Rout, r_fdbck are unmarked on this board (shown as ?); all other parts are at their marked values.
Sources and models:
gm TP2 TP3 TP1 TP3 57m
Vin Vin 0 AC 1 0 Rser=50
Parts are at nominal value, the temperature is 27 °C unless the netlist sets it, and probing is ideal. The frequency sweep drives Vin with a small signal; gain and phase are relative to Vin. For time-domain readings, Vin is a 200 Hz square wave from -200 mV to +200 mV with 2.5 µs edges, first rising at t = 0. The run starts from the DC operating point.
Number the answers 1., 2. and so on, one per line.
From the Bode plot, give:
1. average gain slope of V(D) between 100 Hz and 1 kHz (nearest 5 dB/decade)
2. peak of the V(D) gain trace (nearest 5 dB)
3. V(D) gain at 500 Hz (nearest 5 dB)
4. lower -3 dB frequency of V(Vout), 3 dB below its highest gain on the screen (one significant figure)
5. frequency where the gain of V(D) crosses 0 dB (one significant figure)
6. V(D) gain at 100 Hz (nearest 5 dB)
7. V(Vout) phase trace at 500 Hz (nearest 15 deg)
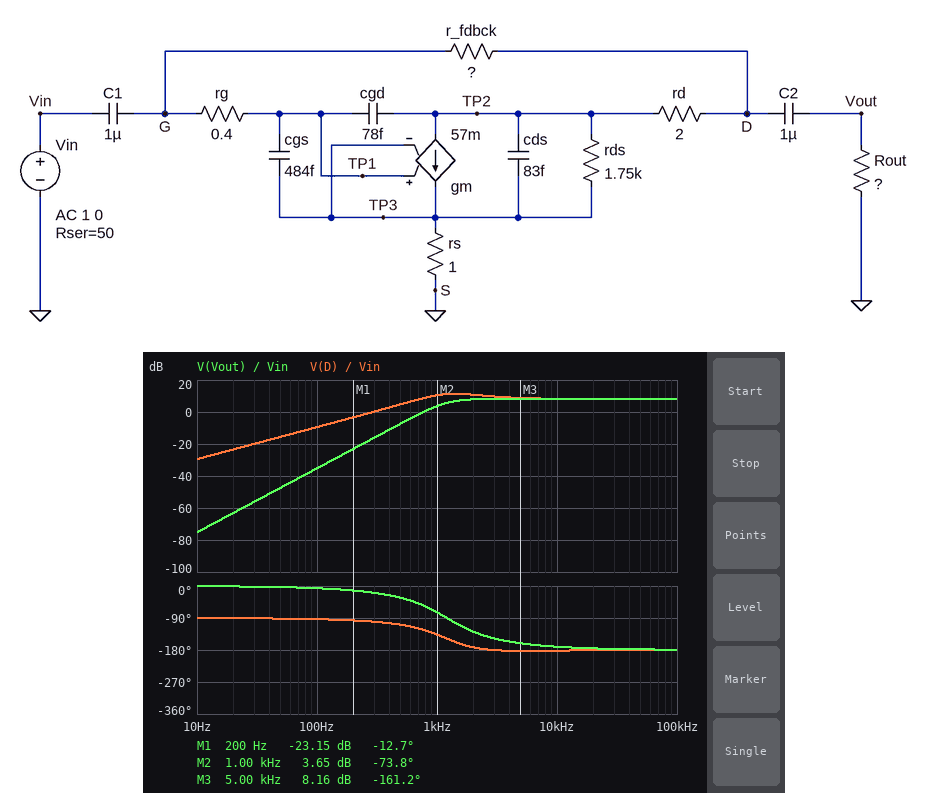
1. 20 dB/decade
2. 10 dB
3. 5 dB
4. 1 kHz
5. 300 Hz
6. -10 dB
7. -30 deg
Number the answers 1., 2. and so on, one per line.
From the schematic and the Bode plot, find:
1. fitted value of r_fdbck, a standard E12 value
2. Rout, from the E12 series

1. 560 Ω
2. 82 Ω
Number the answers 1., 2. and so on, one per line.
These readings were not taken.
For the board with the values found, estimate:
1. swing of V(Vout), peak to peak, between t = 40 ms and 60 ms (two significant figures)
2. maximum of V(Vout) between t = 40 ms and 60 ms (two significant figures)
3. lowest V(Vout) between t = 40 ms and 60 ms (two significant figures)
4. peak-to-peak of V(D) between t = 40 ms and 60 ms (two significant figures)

1. 2.0 V
2. 1.0 V
3. -1.0 V
4. 2.1 V
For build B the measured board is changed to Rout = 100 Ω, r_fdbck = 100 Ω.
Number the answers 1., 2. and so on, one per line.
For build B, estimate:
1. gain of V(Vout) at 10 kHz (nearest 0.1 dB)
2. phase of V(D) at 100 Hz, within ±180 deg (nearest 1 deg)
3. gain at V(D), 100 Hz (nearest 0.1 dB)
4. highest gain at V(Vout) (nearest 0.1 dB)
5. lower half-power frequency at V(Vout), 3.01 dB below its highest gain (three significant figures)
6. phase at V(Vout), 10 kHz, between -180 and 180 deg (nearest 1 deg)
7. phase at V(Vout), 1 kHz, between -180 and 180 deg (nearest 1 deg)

1. -1.8 dB
2. -93 deg
3. -25.9 dB
4. -1.6 dB
5. 2.35 kHz
6. -162 deg
7. -62 deg
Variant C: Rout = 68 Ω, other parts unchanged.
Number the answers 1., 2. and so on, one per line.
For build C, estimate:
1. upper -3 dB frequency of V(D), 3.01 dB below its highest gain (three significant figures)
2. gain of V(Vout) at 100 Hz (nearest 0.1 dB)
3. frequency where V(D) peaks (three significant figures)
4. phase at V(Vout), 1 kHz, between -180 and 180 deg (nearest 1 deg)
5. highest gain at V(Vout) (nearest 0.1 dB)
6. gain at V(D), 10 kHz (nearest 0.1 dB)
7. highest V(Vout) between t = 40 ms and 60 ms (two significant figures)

1. 3.66 kHz
2. -36.8 dB
3. 1.39 kHz
4. -70 deg
5. 7.2 dB
6. 7.3 dB
7. 890 mV
